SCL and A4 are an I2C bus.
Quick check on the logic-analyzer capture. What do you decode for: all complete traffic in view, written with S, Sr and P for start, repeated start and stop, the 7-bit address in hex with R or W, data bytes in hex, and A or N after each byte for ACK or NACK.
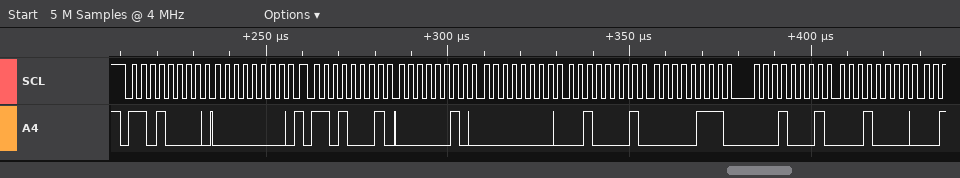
S 68W A 00 A Sr 68R A 02 A 00 A 21 A 07 A 11 A 10 A
